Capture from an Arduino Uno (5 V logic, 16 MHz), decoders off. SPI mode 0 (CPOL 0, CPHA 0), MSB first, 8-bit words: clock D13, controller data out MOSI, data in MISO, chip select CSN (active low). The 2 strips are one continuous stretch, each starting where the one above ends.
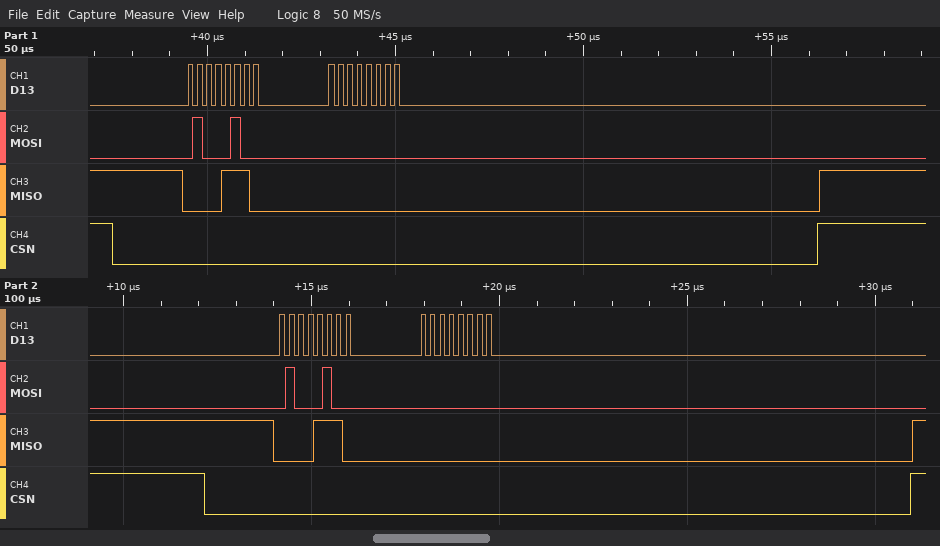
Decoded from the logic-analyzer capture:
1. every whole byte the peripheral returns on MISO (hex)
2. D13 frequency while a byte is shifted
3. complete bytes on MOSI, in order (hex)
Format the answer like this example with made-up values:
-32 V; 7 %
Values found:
0E 00 0E 00; 4 MHz; 44 00 44 00
